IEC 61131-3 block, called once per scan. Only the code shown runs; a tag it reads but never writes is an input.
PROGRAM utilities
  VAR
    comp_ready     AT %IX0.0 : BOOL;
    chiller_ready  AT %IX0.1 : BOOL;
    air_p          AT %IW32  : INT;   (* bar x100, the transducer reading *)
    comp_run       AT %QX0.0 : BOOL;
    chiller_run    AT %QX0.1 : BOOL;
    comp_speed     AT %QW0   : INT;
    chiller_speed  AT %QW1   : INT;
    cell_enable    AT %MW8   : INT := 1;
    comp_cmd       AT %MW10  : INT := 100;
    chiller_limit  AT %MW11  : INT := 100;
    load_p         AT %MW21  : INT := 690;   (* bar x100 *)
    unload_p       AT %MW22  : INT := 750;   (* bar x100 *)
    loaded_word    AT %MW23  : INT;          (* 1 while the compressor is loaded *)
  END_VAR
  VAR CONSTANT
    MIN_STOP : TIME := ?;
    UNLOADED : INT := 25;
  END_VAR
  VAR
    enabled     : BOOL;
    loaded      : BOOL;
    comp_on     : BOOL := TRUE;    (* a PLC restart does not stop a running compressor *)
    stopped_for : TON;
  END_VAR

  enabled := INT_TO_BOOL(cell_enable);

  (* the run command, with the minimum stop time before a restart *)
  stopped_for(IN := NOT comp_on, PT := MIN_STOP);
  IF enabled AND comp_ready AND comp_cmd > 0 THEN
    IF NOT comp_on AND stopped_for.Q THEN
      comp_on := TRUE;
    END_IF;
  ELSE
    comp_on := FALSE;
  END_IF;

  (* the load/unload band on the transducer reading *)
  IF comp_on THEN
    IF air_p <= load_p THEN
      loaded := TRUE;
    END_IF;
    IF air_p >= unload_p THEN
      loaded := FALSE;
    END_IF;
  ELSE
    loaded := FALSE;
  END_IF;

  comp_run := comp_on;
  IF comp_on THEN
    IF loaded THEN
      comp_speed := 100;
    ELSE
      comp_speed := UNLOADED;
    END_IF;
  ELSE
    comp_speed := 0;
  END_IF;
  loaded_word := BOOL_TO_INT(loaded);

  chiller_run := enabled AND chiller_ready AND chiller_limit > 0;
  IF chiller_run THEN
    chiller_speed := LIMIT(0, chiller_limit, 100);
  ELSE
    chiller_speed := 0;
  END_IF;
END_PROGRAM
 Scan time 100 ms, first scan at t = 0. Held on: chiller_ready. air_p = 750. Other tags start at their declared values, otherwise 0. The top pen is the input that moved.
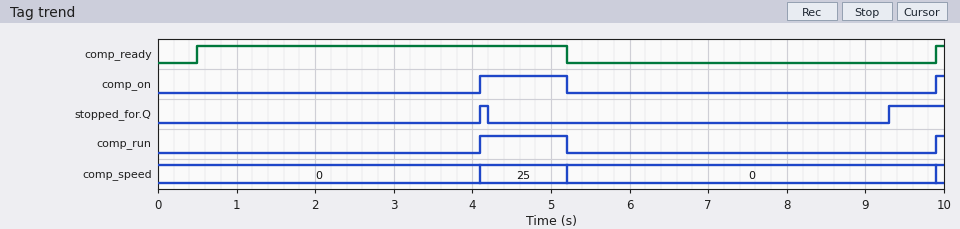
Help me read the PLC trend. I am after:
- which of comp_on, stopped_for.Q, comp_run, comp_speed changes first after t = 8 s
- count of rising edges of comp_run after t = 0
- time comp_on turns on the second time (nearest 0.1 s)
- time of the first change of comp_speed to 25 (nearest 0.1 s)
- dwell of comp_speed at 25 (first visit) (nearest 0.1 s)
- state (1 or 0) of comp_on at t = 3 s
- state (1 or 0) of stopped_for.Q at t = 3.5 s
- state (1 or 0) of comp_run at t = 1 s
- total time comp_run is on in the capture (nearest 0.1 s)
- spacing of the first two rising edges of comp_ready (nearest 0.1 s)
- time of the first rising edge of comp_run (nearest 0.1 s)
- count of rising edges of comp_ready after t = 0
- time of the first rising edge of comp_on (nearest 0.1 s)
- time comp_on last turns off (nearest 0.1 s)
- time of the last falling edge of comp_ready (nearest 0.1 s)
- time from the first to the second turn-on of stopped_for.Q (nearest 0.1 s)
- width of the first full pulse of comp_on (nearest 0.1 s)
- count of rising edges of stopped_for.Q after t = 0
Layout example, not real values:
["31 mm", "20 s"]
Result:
["stopped_for.Q", "2", "9.9 s", "4.1 s", "1.1 s", "0", "0", "0", "1.2 s", "9.4 s", "4.1 s", "2", "4.1 s", "5.2 s", "5.2 s", "5.2 s", "1.1 s", "2"]
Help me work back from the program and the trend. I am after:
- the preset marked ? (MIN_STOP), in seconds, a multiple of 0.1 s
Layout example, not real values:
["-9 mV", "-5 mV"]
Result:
["4.0 s"]
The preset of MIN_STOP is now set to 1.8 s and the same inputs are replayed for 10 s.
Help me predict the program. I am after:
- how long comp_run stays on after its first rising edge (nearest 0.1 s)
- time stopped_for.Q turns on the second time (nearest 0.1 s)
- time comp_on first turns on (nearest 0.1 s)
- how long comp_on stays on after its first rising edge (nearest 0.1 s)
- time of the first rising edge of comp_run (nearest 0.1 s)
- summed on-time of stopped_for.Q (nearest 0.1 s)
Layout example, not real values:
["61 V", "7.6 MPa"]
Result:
["3.3 s", "7.1 s", "1.9 s", "3.3 s", "1.9 s", "3.0 s"]
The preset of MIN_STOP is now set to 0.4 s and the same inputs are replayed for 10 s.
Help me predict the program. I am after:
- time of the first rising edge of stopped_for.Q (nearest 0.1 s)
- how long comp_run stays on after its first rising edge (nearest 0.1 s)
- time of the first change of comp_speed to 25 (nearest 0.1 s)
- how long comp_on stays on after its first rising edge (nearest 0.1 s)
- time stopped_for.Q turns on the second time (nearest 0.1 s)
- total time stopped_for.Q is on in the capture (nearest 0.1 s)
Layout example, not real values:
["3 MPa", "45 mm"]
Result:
["0.5 s", "4.7 s", "0.5 s", "4.7 s", "5.7 s", "4.4 s"]
